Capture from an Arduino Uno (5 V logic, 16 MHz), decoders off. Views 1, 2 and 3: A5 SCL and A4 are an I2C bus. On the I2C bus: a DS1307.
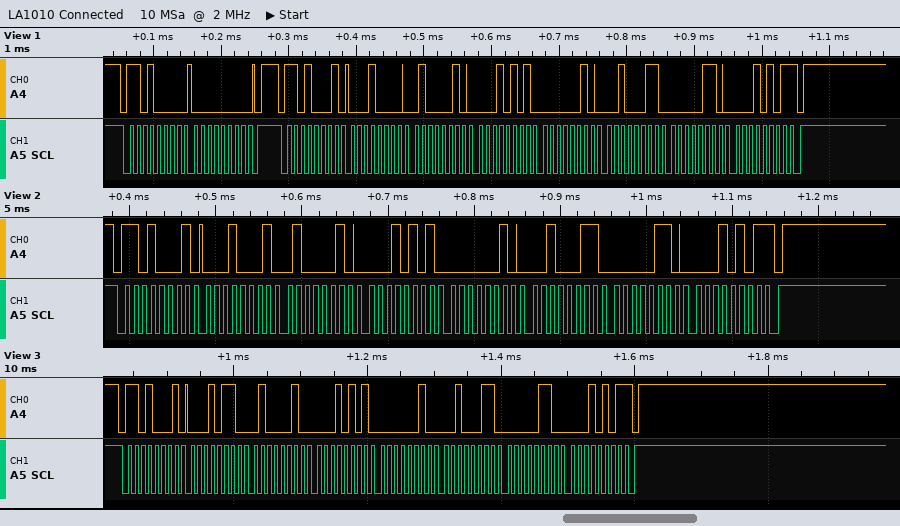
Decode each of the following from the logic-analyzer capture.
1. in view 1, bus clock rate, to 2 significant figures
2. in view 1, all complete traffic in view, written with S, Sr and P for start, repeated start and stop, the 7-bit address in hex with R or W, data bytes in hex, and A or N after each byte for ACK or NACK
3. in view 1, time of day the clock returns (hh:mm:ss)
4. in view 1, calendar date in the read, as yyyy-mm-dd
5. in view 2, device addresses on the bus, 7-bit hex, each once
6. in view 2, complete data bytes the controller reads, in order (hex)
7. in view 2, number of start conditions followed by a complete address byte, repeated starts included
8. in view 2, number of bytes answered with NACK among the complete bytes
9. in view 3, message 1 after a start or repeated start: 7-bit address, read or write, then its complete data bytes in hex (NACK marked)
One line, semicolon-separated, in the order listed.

100 kHz; S 68W A 00 A P S 68R A 10 A 42 A 15 A 02 A 23 A 06 A 15 N P; 15:42:10; 2015-06-23; 0x68; 11 42 15 02 23 06 15; 1; 1; 0x68 read: 16 42 15 02 23 06 15 NACK
